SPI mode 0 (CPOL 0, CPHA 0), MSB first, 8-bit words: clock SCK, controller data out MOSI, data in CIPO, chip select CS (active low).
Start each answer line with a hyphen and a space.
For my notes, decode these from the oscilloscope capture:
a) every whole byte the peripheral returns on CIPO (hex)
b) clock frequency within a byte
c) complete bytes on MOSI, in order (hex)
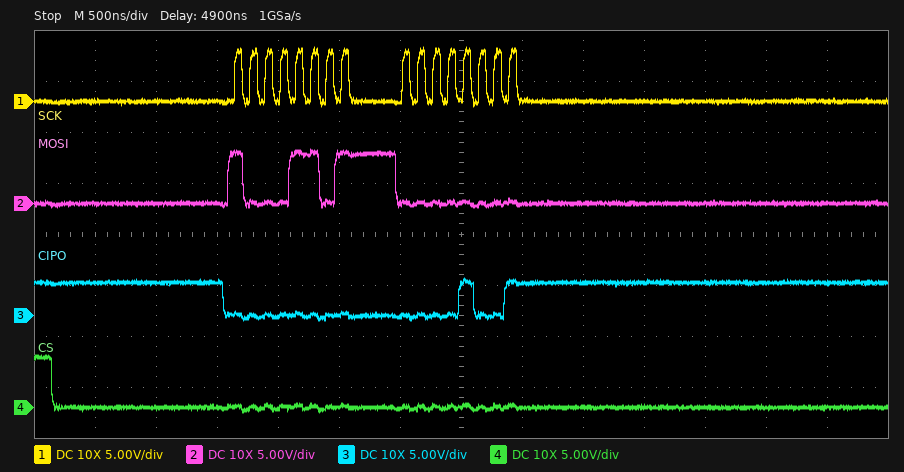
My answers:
- 0x00 0x09
- 8 MHz
- 0x8D 0x00
